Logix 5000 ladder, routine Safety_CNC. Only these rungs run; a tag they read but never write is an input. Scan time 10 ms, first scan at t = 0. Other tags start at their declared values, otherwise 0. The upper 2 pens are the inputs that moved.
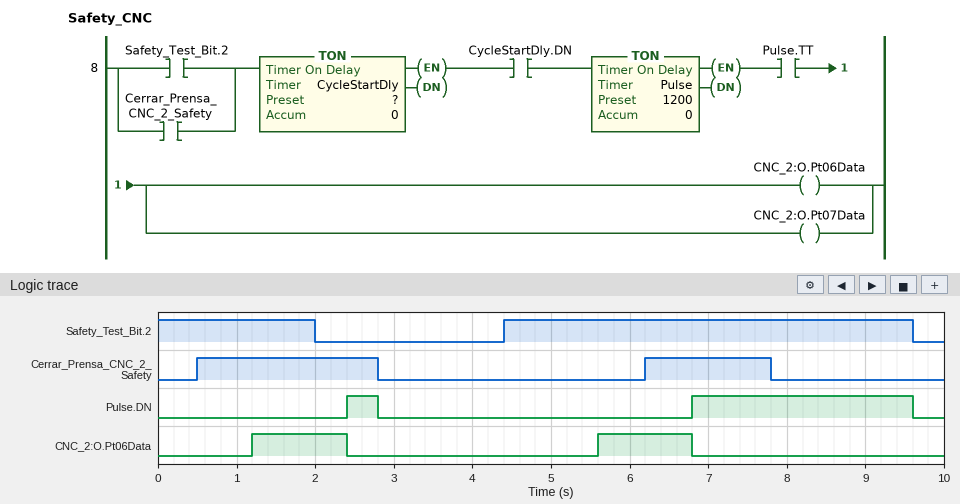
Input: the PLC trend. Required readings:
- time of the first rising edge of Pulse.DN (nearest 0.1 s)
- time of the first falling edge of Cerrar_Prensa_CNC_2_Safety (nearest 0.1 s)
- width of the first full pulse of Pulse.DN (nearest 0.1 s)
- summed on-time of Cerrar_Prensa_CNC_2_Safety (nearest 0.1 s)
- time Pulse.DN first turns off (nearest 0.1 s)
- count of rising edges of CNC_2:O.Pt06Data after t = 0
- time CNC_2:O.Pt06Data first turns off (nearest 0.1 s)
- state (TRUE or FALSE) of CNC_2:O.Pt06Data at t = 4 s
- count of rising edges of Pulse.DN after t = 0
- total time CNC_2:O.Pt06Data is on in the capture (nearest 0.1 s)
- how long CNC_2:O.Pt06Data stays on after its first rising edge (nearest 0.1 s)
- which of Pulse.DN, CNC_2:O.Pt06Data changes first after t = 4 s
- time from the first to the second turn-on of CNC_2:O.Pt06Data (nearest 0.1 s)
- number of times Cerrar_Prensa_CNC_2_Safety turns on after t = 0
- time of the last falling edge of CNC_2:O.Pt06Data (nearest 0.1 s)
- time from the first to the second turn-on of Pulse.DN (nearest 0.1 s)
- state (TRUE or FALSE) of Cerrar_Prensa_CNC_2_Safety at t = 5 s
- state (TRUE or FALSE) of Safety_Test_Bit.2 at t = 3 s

2.4 s
2.8 s
0.4 s
3.9 s
2.8 s
2
2.4 s
FALSE
2
2.4 s
1.2 s
CNC_2:O.Pt06Data
4.4 s
2
6.8 s
4.4 s
FALSE
FALSE
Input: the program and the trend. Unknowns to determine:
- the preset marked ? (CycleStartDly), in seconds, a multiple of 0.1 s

1.2 s
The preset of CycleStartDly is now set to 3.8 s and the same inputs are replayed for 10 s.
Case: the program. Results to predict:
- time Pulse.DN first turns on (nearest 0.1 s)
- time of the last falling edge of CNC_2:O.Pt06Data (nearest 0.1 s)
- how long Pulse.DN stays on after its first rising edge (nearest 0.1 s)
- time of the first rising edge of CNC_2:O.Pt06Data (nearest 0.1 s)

9.4 s
9.4 s
0.2 s
8.2 s
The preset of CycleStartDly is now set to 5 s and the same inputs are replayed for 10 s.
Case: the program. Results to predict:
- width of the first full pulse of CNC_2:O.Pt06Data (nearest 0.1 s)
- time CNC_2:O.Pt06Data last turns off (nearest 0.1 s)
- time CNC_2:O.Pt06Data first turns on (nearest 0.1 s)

0.2 s
9.6 s
9.4 s
